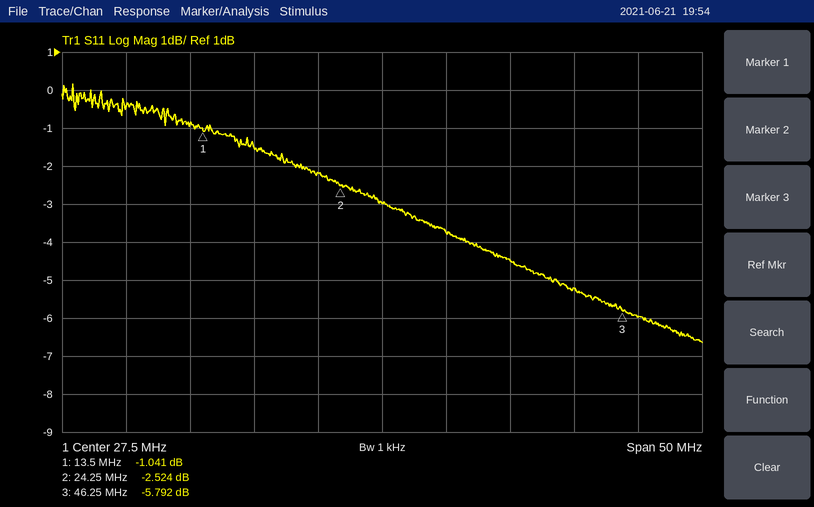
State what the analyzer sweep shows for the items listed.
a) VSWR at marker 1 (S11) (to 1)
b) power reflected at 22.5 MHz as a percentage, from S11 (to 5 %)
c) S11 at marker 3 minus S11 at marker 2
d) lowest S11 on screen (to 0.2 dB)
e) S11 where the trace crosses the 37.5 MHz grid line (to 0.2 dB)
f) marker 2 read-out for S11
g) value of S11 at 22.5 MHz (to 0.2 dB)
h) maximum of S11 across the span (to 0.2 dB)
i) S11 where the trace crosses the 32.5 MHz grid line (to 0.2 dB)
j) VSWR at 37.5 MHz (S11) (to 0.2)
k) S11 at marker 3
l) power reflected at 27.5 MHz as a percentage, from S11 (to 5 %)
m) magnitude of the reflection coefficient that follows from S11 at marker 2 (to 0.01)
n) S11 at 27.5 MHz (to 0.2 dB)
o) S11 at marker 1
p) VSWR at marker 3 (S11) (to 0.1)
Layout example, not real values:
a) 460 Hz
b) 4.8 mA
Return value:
a) 17
b) 60 %
c) -3.268 dB
d) -6.6 dB
e) -4.4 dB
f) -2.524 dB
g) -2.2 dB
h) 0.2 dB
i) -3.8 dB
j) 4.0
k) -5.792 dB
l) 50 %
m) 0.75
n) -3.0 dB
o) -1.041 dB
p) 3.1
